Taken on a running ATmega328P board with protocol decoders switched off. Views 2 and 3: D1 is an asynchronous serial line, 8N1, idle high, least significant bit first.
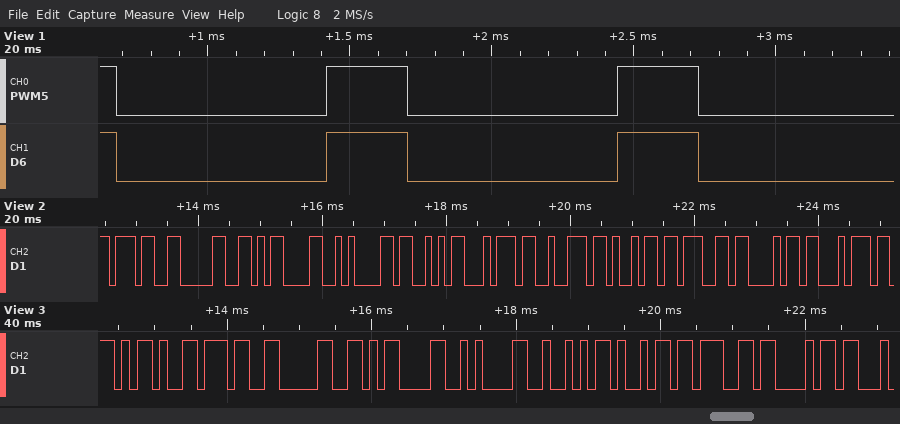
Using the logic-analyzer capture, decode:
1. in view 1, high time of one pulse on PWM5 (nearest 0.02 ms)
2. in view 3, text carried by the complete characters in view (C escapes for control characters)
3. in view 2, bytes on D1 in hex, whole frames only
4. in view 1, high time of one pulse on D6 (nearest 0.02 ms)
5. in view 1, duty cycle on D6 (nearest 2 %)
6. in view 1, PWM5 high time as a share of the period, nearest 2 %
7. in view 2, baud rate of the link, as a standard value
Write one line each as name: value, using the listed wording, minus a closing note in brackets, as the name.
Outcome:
in view 1, high time of one pulse on PWM5: 0.28 ms
in view 3, text carried by the complete characters in view: "-70\r\nRigh"
in view 2, bytes on D1 in hex, whole frames only: 37 30 0D 0A 53 74 72 69 67 68 74
in view 1, high time of one pulse on D6: 0.28 ms
in view 1, duty cycle on D6: 28 %
in view 1, PWM5 high time as a share of the period, nearest 2 %: 28 %
in view 2, baud rate of the link, as a standard value: 9600 baud
